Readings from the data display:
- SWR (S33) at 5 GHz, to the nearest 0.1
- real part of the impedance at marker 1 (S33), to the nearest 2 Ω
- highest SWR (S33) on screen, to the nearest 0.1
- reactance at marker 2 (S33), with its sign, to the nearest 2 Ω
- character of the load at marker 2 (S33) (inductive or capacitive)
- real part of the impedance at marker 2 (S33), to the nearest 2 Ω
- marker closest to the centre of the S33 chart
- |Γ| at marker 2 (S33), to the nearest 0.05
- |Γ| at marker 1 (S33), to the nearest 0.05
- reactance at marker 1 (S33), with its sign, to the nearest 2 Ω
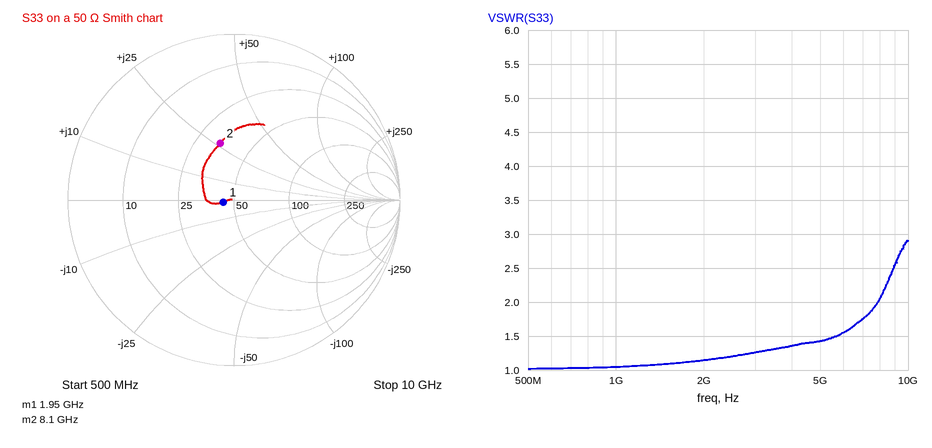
1.4
44 Ω
2.9
+26 Ω
inductive
34 Ω
marker 1
0.35
0.05
-2 Ω
